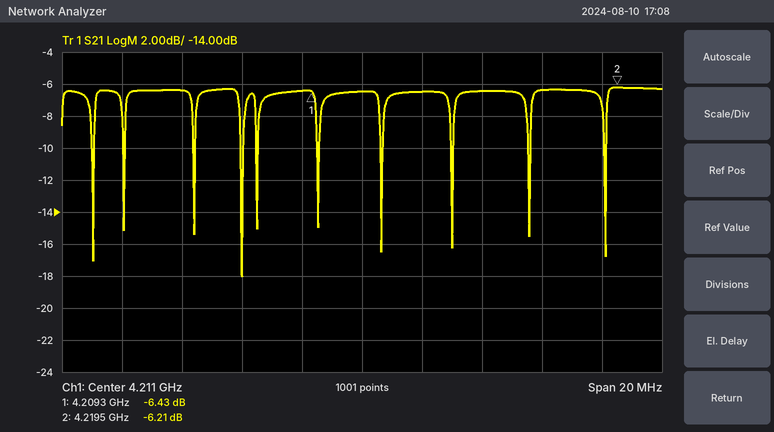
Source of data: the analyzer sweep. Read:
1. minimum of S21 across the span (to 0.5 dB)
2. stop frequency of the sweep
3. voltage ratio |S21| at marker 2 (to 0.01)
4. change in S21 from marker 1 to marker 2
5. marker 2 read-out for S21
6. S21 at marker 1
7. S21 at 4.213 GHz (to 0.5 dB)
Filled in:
-18.0 dB
4.221 GHz
0.49
0.22 dB
-6.21 dB
-6.43 dB
-6.5 dB
